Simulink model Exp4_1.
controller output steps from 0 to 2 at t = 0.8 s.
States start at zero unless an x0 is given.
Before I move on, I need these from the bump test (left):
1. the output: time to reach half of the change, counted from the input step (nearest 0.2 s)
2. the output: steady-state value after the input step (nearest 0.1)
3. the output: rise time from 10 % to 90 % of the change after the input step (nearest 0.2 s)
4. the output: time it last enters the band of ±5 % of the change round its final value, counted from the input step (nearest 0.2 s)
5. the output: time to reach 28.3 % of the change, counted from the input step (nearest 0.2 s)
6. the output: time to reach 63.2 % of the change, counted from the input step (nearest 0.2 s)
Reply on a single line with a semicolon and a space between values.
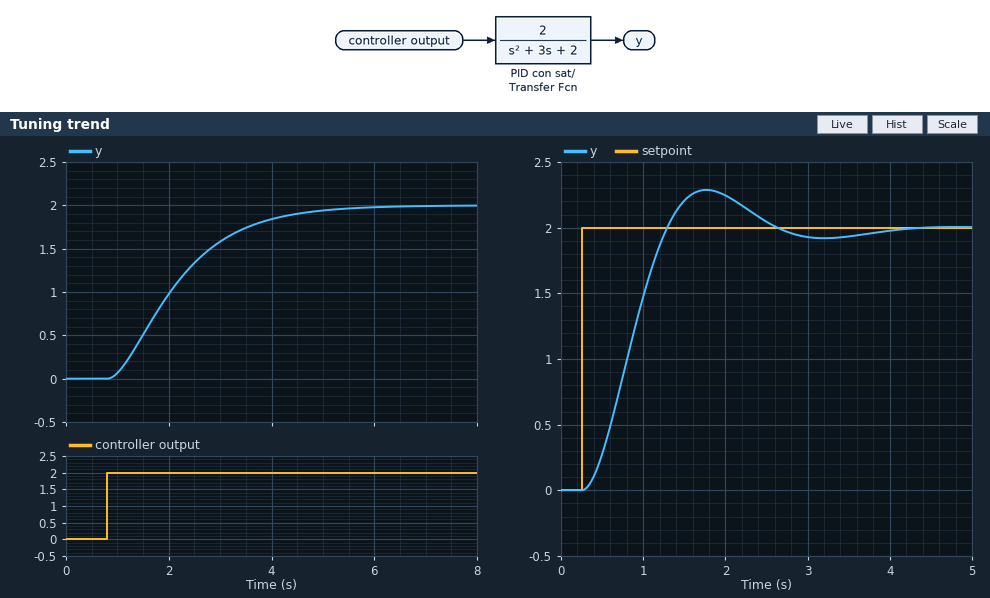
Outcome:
1.2 s; 2.0; 2.6 s; 3.6 s; 0.8 s; 1.6 s
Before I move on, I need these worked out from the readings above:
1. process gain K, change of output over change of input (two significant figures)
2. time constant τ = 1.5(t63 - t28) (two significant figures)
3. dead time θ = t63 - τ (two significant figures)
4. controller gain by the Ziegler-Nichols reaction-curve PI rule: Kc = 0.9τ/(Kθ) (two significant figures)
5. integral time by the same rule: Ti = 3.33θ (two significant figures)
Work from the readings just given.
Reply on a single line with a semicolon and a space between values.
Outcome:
1.0; 1.2 s; 0.40 s; 2.7; 1.3 s
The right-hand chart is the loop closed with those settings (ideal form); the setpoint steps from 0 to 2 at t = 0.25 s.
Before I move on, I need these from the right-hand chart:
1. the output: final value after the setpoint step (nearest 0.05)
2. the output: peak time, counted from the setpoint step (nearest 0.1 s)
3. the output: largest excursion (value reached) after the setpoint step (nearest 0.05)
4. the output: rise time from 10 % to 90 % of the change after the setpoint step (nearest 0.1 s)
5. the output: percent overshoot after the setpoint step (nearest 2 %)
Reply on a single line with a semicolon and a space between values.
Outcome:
2.00; 1.5 s; 2.30; 0.7 s; 14 %
